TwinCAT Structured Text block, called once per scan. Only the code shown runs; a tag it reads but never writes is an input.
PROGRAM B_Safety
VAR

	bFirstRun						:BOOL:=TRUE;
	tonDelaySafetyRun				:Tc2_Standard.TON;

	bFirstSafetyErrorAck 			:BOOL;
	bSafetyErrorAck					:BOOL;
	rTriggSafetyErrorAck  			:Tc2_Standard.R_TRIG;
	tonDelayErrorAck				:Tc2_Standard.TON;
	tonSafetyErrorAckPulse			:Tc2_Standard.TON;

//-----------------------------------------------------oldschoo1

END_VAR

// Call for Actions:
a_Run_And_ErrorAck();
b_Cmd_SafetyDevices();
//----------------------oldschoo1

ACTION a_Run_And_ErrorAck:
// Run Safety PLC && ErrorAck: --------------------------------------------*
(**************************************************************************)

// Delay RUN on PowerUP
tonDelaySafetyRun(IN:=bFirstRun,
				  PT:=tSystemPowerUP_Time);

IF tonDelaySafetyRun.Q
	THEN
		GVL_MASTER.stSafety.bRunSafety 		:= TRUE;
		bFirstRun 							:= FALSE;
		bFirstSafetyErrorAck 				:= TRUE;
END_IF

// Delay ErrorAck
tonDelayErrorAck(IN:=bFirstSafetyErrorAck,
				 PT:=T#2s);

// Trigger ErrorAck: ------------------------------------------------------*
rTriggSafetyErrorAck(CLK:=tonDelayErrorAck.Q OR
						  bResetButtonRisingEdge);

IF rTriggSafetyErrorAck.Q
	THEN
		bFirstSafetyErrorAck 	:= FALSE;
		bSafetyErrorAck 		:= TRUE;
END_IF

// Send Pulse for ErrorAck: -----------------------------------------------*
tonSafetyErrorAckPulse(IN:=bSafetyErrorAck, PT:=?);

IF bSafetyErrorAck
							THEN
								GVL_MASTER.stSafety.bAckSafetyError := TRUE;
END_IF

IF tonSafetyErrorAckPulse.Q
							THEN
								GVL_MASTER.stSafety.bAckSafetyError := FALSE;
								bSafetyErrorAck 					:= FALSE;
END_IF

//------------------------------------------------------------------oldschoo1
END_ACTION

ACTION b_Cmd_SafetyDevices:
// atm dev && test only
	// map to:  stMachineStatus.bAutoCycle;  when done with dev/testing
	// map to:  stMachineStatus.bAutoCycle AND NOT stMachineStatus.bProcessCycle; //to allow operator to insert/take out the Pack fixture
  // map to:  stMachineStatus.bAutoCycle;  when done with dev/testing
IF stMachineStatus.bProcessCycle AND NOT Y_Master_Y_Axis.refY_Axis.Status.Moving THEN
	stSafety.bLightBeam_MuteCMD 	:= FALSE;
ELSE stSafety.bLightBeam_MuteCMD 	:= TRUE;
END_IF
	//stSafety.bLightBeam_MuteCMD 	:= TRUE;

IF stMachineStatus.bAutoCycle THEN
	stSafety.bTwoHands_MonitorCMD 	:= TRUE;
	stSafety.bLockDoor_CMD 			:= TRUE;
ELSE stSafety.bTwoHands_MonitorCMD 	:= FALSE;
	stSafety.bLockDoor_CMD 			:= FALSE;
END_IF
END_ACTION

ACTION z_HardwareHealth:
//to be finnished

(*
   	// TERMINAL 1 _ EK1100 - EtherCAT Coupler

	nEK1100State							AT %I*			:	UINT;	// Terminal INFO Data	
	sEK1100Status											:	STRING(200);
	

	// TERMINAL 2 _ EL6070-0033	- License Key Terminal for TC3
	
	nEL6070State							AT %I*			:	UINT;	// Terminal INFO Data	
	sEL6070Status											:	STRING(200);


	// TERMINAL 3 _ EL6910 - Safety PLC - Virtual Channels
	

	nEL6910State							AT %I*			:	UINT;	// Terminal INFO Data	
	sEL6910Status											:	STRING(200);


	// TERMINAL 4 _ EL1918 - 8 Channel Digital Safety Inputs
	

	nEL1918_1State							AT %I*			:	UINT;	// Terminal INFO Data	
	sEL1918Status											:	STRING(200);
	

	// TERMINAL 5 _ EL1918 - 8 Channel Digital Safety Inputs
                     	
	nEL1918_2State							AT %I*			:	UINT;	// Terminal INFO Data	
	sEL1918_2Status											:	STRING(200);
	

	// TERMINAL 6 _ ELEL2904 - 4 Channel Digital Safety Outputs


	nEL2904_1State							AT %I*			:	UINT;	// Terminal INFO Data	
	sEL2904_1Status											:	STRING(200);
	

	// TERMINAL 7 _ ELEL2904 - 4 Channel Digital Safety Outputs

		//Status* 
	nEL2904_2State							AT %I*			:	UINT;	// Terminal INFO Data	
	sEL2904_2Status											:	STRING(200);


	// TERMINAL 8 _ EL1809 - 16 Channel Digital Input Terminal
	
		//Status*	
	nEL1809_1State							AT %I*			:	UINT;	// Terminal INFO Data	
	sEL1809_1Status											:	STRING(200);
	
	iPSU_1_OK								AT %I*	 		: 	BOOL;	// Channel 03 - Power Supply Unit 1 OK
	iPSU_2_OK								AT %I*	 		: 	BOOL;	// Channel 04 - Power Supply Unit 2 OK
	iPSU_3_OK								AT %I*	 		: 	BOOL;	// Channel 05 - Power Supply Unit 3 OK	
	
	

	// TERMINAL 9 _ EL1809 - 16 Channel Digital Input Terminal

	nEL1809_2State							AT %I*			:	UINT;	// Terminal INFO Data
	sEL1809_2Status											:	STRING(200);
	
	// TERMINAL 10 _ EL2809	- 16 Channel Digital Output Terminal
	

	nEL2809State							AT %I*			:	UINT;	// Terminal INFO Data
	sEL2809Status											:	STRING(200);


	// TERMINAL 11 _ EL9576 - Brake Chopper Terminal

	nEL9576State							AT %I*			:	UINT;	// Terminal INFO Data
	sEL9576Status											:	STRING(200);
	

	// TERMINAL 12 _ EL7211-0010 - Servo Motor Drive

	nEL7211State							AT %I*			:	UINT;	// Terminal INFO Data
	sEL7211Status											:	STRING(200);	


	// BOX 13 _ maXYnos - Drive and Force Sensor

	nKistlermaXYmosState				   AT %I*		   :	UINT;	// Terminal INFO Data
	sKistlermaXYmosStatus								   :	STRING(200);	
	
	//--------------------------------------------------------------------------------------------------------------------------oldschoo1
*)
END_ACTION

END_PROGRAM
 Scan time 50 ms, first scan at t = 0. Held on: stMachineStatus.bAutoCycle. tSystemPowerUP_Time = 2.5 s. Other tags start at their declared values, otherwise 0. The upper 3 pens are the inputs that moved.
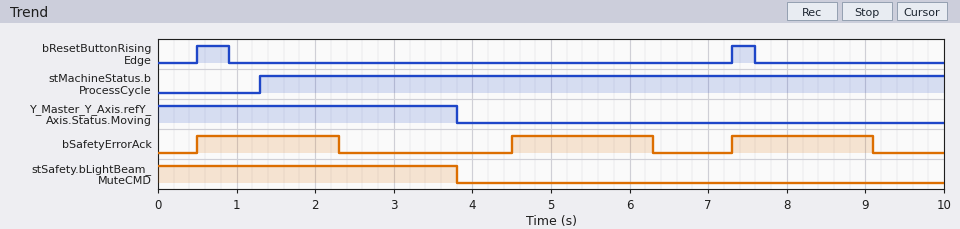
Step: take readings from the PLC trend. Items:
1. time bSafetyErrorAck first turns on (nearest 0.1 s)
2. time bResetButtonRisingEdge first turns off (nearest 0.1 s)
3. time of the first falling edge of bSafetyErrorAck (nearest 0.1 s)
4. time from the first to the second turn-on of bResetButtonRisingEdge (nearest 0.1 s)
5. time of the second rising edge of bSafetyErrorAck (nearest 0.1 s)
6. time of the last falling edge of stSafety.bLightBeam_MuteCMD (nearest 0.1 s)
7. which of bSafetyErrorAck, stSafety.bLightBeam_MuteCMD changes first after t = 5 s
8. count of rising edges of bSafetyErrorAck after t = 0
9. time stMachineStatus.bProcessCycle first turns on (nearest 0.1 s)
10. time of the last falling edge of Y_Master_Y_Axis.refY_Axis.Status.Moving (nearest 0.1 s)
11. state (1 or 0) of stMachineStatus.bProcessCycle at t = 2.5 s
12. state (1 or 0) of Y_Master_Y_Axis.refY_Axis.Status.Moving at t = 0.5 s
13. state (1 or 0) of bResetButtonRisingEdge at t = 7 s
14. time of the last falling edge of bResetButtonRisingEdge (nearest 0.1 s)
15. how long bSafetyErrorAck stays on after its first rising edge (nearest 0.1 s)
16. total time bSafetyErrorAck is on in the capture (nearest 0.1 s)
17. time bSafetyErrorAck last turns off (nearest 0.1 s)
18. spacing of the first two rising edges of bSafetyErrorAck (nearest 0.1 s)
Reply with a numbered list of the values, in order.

1. 0.5 s
2. 0.9 s
3. 2.3 s
4. 6.8 s
5. 4.5 s
6. 3.8 s
7. bSafetyErrorAck
8. 3
9. 1.3 s
10. 3.8 s
11. 1
12. 1
13. 0
14. 7.6 s
15. 1.8 s
16. 5.4 s
17. 9.1 s
18. 4.0 s
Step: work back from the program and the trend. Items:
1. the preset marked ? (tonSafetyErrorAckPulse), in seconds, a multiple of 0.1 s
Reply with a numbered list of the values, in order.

1. 1.8 s
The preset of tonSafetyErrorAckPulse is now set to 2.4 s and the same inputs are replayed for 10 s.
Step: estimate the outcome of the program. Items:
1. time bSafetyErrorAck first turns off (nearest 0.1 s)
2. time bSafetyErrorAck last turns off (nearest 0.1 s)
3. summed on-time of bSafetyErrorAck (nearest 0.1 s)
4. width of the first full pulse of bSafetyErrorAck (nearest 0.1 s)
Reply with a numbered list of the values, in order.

1. 2.9 s
2. 9.7 s
3. 7.2 s
4. 2.4 s
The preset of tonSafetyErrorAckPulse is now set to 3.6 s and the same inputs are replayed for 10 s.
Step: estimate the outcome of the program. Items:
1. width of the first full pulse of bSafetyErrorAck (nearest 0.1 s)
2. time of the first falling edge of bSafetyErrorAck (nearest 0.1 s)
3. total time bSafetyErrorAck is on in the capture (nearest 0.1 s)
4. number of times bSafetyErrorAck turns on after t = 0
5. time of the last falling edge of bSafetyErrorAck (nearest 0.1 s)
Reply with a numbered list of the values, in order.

1. 3.6 s
2. 4.1 s
3. 7.2 s
4. 2
5. 8.1 s
